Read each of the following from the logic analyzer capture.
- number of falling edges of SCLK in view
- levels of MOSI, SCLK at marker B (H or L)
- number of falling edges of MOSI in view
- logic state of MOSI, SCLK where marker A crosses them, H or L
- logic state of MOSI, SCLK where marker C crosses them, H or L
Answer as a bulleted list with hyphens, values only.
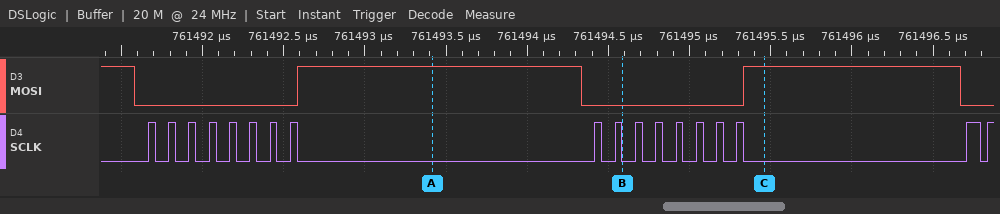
- 17
- MOSI=L, SCLK=L
- 3
- MOSI=H, SCLK=L
- MOSI=H, SCLK=L
